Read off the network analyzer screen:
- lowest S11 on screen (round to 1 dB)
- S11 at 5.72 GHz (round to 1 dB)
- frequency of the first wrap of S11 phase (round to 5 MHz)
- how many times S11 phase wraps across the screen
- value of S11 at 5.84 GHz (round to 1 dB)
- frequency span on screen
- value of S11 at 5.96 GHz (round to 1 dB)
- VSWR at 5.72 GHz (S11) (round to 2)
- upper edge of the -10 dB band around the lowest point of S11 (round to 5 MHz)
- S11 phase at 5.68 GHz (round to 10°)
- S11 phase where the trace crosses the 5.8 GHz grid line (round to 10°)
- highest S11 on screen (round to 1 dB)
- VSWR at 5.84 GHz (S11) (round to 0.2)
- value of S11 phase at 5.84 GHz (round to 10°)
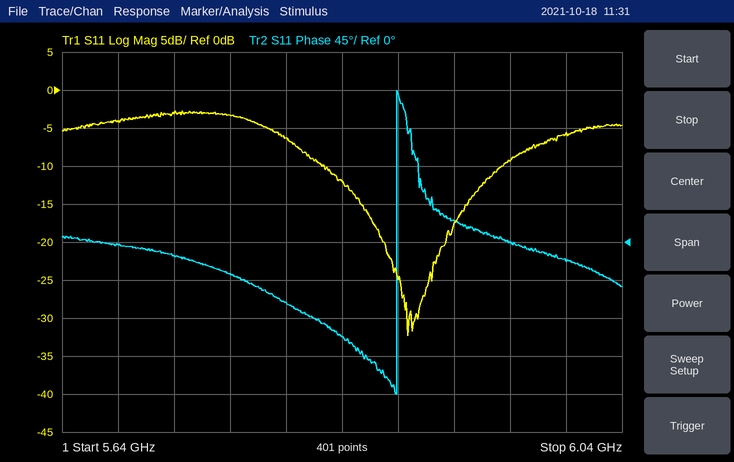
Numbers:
-32 dB
-3 dB
5.880 GHz
1
-12 dB
400 MHz
-9 dB
6
5.955 GHz
0°
-70°
-3 dB
1.6
-110°
